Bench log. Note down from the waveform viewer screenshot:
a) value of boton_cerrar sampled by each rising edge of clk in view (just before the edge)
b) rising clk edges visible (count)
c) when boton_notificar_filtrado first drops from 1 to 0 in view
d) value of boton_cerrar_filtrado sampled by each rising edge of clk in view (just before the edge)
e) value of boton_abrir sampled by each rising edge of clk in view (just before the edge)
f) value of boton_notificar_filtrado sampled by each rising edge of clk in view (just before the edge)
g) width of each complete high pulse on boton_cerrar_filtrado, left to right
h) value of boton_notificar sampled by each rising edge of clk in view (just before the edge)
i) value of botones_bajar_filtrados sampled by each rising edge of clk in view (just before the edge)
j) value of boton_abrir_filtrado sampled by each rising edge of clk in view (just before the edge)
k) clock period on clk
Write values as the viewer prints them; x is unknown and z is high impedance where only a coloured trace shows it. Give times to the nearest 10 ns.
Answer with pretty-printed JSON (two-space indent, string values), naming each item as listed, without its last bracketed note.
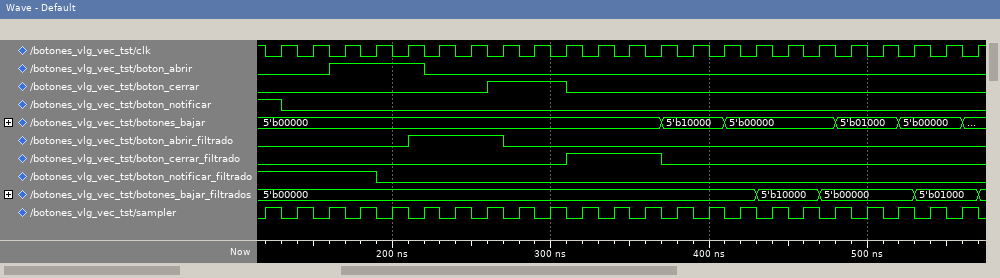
{
  "value of boton_cerrar sampled by each rising edge of clk in view": "0 0 0 0 0 0 0 1 1 1 0 0 0 0 0 0 0 0 0 0 0 0 0",
  "rising clk edges visible": "23",
  "when boton_notificar_filtrado first drops from 1 to 0 in view": "190 ns",
  "value of boton_cerrar_filtrado sampled by each rising edge of clk in view": "0 0 0 0 0 0 0 0 0 0 1 1 1 0 0 0 0 0 0 0 0 0 0",
  "value of boton_abrir sampled by each rising edge of clk in view": "0 0 1 1 1 0 0 0 0 0 0 0 0 0 0 0 0 0 0 0 0 0 0",
  "value of boton_notificar_filtrado sampled by each rising edge of clk in view": "1 1 1 1 0 0 0 0 0 0 0 0 0 0 0 0 0 0 0 0 0 0 0",
  "width of each complete high pulse on boton_cerrar_filtrado, left to right": "60 ns",
  "value of boton_notificar sampled by each rising edge of clk in view": "1 0 0 0 0 0 0 0 0 0 0 0 0 0 0 0 0 0 0 0 0 0 0",
  "value of botones_bajar_filtrados sampled by each rising edge of clk in view": "5'b00000, 5'b00000, 5'b00000, 5'b00000, 5'b00000, 5'b00000, 5'b00000, 5'b00000, 5'b00000, 5'b00000, 5'b00000, 5'b00000, 5'b00000, 5'b00000, 5'b00000, 5'b00000, 5'b10000, 5'b10000, 5'b00000, 5'b00000, 5'b00000, 5'b01000, 5'b01000",
  "value of boton_abrir_filtrado sampled by each rising edge of clk in view": "0 0 0 0 0 1 1 1 0 0 0 0 0 0 0 0 0 0 0 0 0 0 0",
  "clock period on clk": "20 ns"
}
